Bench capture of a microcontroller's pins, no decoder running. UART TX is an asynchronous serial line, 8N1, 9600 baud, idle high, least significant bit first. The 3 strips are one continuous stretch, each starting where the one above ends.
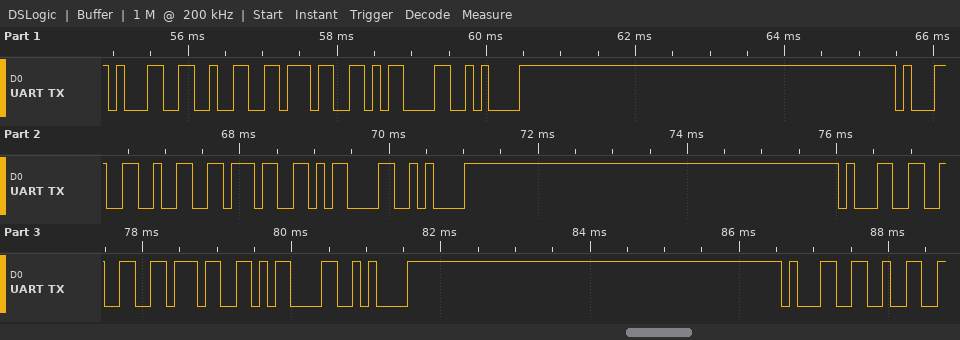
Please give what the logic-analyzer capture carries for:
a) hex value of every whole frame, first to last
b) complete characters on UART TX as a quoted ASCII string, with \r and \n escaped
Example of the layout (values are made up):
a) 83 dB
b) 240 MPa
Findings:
a) 0x31 0x32 0x37 0x0D 0x0A 0x31 0x32 0x37 0x0D 0x0A 0x31 0x32 0x37 0x0D 0x0A 0x31 0x32
b) "127\r\n127\r\n127\r\n12"
